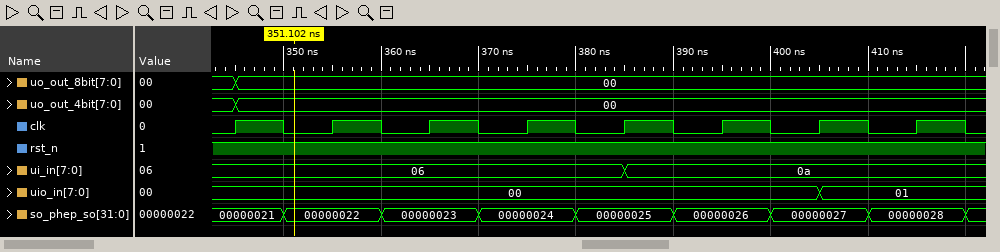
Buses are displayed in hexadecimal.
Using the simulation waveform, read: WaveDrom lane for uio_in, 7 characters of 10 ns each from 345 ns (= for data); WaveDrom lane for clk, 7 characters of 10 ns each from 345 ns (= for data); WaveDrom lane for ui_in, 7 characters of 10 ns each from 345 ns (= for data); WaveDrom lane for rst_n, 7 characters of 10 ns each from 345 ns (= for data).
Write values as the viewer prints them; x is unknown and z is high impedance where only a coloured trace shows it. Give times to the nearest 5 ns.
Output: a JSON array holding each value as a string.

["{name: 'uio_in', wave: '=.....=', data: '00 01'}", "{name: 'clk', wave: 'p......'}", "{name: 'ui_in', wave: '=...=..', data: '06 0a'}", "{name: 'rst_n', wave: '1......'}"]
